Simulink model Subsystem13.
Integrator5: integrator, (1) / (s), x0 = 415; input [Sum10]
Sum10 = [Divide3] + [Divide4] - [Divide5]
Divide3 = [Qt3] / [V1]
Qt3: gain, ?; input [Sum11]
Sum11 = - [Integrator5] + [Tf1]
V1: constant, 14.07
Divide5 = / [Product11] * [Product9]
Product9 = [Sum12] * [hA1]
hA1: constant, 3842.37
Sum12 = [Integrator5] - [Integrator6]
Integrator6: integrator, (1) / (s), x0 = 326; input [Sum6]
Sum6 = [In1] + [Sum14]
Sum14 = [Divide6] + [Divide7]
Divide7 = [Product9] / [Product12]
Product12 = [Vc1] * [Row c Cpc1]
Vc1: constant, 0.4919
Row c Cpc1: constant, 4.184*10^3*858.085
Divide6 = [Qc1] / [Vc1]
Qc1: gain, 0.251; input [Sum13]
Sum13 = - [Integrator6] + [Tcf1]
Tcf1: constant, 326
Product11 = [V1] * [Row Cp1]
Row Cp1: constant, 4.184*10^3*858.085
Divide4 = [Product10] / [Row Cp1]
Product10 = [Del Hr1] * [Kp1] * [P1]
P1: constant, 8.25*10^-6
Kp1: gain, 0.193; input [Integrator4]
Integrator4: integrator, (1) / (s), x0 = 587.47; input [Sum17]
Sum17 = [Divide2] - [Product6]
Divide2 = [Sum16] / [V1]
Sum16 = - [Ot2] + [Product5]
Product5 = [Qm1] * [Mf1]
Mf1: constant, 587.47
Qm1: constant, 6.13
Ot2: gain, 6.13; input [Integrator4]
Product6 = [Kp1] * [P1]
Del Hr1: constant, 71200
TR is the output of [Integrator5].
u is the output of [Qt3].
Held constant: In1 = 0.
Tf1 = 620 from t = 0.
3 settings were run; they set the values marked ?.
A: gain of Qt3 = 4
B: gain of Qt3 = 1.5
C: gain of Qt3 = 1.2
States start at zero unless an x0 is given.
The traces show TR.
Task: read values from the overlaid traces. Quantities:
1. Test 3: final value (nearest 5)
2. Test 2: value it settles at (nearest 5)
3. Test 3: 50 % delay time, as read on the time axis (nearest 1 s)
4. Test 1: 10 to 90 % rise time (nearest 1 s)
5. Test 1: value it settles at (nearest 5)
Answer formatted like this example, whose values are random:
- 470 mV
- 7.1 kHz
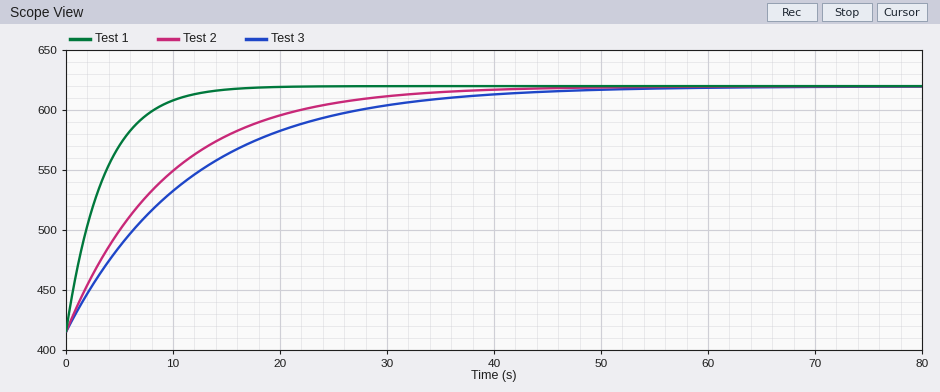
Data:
- 620
- 620
- 8 s
- 8 s
- 620
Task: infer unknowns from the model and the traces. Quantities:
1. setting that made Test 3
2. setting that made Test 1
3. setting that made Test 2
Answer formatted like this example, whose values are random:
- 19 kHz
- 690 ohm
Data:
- C
- A
- B
